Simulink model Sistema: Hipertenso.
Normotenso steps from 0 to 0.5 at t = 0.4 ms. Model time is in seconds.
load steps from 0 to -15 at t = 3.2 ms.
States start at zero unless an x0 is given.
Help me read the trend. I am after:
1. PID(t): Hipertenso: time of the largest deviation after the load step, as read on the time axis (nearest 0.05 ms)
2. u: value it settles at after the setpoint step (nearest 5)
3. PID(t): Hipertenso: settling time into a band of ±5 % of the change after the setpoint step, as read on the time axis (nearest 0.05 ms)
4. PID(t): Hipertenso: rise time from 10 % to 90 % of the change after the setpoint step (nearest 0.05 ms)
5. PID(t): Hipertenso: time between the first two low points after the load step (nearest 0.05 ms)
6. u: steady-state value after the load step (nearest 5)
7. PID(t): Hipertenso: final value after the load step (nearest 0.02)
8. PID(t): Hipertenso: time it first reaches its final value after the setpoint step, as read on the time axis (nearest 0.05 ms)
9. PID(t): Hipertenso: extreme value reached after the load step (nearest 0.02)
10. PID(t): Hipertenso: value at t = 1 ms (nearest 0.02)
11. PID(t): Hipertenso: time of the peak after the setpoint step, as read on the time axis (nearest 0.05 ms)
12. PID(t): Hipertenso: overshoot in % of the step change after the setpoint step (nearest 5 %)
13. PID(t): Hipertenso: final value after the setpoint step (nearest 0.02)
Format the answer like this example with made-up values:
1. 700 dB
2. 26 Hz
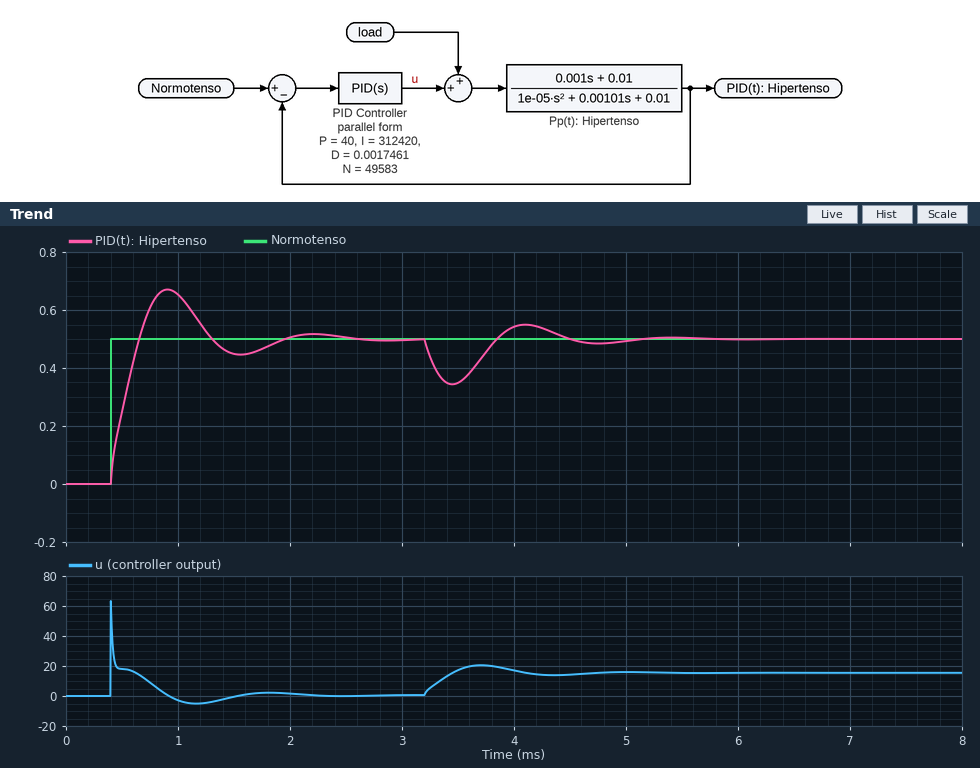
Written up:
1. 3.45 ms
2. 0
3. 1.80 ms
4. 0.20 ms
5. 1.30 ms
6. 15
7. 0.50
8. 0.65 ms
9. 0.34
10. 0.66
11. 0.90 ms
12. 35 %
13. 0.50
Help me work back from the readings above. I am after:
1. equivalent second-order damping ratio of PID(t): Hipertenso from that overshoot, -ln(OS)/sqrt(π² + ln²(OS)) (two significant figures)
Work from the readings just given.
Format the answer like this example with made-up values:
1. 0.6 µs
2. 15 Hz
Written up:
1. 0.32
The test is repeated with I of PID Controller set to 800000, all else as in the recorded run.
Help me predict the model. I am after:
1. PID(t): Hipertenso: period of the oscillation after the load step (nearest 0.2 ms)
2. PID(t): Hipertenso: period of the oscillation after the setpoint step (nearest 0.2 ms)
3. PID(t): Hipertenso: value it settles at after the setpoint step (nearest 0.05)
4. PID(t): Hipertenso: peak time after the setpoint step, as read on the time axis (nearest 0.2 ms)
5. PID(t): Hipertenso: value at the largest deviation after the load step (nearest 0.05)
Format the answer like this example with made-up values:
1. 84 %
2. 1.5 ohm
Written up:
1. 0.8 ms
2. 0.8 ms
3. 0.50
4. 0.8 ms
5. 0.40
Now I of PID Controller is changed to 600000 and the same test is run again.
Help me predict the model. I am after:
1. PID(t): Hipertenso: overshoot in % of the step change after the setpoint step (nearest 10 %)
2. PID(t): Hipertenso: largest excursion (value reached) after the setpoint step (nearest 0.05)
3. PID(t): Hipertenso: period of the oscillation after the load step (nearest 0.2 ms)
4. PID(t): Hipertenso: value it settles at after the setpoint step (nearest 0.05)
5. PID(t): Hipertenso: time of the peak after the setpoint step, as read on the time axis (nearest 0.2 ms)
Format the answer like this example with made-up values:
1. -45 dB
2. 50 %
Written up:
1. 40 %
2. 0.70
3. 1.0 ms
4. 0.50
5. 0.8 ms
